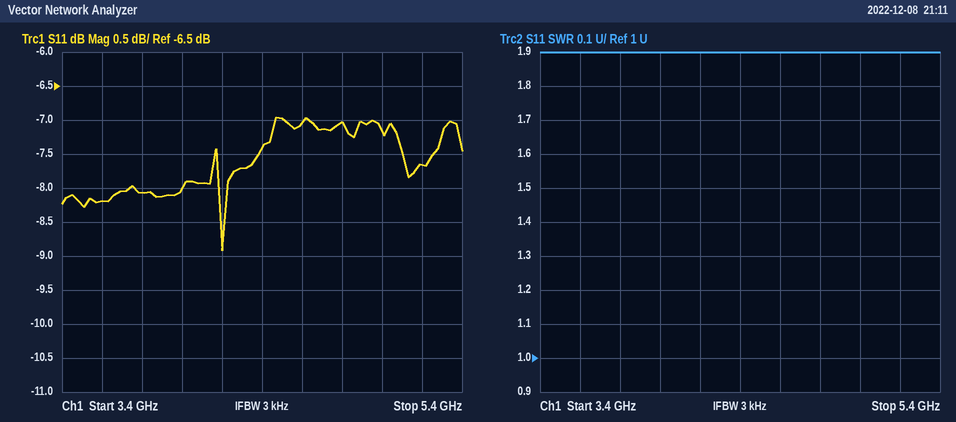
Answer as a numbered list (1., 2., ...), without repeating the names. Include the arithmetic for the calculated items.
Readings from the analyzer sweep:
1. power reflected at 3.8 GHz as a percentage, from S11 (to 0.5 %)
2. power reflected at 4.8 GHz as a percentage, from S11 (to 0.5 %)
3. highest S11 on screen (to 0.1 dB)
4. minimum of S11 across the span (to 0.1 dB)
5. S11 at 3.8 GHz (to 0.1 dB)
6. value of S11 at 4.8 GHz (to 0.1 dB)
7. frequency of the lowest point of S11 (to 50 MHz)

1. 10^(-8.1/10) ≈ 15.5 %
2. 10^(-7/10) ≈ 20.0 %
3. -7.0 dB
4. -8.9 dB
5. -8.1 dB
6. -7.0 dB
7. 4.20 GHz
